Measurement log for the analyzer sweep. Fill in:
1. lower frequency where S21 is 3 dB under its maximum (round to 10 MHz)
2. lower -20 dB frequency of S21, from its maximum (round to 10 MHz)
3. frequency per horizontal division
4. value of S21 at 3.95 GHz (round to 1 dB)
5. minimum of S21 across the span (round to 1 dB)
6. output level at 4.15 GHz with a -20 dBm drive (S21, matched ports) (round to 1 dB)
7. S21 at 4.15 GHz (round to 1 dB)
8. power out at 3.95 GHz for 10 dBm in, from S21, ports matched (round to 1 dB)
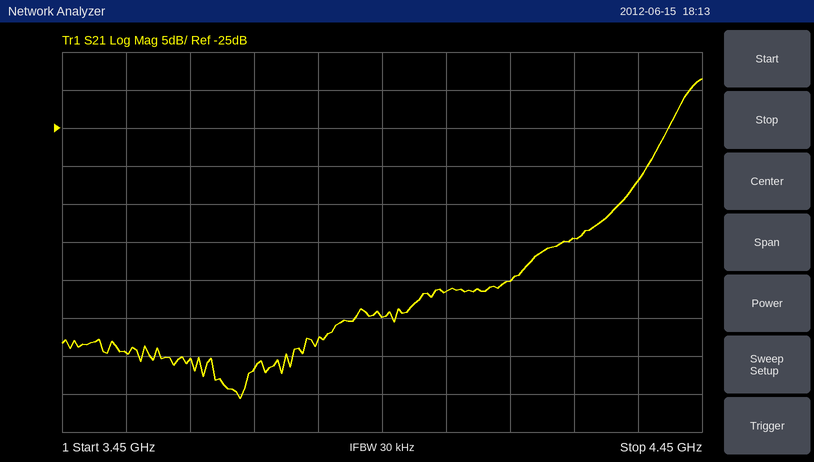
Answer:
4.42 GHz
4.27 GHz
100 MHz
-50 dB
-61 dB
-65 dBm
-45 dB
-40 dBm
